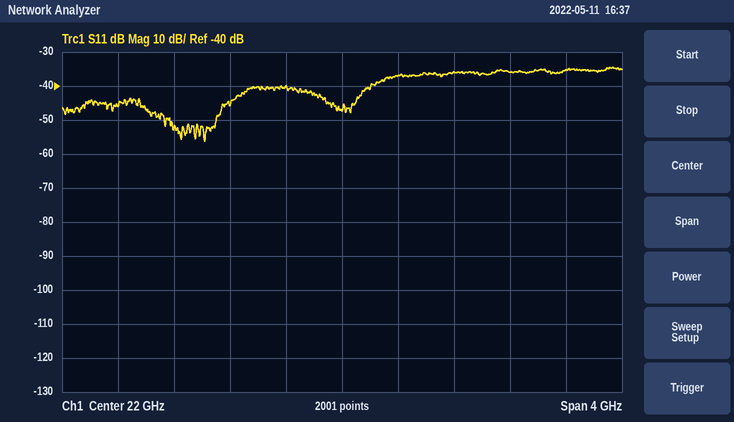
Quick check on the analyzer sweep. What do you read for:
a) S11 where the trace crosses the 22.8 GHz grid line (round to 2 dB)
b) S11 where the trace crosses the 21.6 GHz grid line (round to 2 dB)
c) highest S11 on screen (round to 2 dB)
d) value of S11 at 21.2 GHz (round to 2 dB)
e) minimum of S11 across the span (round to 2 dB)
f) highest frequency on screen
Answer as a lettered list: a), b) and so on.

a) -36 dB
b) -40 dB
c) -34 dB
d) -46 dB
e) -56 dB
f) 24 GHz
